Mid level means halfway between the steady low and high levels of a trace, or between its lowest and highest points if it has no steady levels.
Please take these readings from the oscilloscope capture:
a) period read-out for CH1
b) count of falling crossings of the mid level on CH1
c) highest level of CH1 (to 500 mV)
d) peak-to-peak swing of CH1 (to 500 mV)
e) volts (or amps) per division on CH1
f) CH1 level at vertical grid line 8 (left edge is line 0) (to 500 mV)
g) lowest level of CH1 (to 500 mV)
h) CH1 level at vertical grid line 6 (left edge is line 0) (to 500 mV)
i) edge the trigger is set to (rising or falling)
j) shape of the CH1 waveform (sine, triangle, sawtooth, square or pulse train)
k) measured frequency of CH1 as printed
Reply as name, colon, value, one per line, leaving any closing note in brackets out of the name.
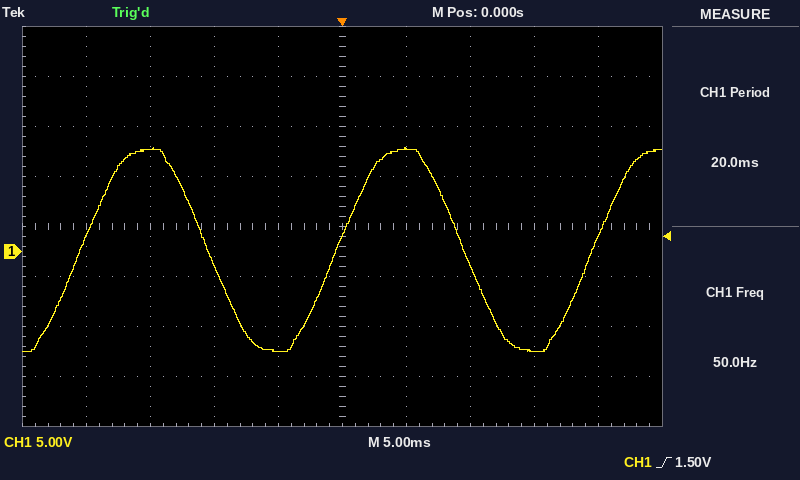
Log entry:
period read-out for CH1: 20.0 ms
count of falling crossings of the mid level on CH1: 2
highest level of CH1: 10.5 V
peak-to-peak swing of CH1: 20.5 V
volts (or amps) per division on CH1: 5 V
CH1 level at vertical grid line 8 (left edge is line 0): -10.0 V
lowest level of CH1: -10.0 V
CH1 level at vertical grid line 6 (left edge is line 0): 10.5 V
edge the trigger is set to: rising
shape of the CH1 waveform: sine
measured frequency of CH1 as printed: 50.0 Hz
